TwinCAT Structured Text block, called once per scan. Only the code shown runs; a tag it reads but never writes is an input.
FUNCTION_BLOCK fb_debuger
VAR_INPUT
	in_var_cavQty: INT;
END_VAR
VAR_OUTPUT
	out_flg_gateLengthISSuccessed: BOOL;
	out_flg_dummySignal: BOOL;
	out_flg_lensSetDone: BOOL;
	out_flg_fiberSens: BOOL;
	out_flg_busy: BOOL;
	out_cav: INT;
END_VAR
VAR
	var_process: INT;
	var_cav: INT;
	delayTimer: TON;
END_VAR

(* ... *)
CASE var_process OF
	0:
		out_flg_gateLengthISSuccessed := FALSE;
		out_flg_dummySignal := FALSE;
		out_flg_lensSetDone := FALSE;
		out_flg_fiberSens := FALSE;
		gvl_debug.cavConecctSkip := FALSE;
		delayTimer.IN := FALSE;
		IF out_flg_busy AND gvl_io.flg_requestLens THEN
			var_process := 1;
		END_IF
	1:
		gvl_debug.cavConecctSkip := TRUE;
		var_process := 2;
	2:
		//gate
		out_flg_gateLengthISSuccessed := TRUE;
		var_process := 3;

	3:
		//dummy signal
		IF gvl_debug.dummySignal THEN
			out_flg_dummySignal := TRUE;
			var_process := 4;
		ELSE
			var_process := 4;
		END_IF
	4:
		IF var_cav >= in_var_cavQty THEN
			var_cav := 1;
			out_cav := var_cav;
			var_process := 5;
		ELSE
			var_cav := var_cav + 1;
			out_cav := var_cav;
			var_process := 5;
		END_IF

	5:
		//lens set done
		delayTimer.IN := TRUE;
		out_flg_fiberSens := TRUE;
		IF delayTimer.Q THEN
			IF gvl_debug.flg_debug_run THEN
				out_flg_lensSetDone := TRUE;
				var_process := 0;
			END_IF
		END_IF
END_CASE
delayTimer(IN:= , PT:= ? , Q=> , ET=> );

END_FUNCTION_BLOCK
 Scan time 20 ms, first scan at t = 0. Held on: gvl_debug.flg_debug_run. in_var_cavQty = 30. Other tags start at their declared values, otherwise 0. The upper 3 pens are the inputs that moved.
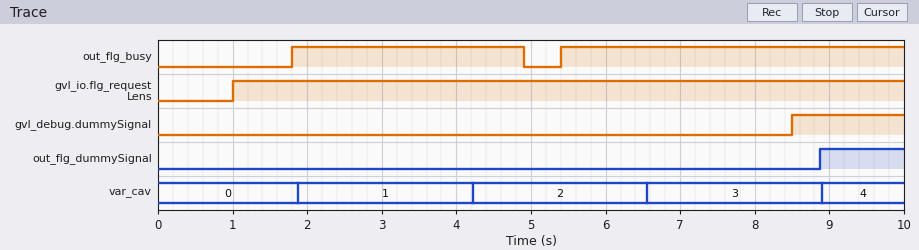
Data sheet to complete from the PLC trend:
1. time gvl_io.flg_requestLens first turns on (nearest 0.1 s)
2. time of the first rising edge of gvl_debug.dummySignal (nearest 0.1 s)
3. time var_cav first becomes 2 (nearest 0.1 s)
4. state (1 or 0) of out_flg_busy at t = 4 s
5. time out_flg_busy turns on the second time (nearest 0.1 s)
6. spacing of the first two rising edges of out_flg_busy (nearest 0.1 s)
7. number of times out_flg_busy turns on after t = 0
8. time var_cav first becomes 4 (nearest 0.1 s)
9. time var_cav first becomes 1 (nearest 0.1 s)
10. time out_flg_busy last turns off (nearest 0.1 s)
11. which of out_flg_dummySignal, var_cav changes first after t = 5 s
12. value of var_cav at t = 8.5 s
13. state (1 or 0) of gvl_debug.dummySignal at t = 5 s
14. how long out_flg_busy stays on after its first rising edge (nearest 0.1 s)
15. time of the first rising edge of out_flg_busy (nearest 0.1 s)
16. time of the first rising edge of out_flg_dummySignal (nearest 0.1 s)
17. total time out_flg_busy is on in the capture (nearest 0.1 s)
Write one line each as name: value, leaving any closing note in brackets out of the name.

time gvl_io.flg_requestLens first turns on: 1.0 s
time of the first rising edge of gvl_debug.dummySignal: 8.5 s
time var_cav first becomes 2: 4.2 s
state (1 or 0) of out_flg_busy at t = 4 s: 1
time out_flg_busy turns on the second time: 5.4 s
spacing of the first two rising edges of out_flg_busy: 3.6 s
number of times out_flg_busy turns on after t = 0: 2
time var_cav first becomes 4: 8.9 s
time var_cav first becomes 1: 1.9 s
time out_flg_busy last turns off: 4.9 s
which of out_flg_dummySignal, var_cav changes first after t = 5 s: var_cav
value of var_cav at t = 8.5 s: 3
state (1 or 0) of gvl_debug.dummySignal at t = 5 s: 0
how long out_flg_busy stays on after its first rising edge: 3.1 s
time of the first rising edge of out_flg_busy: 1.8 s
time of the first rising edge of out_flg_dummySignal: 8.9 s
total time out_flg_busy is on in the capture: 7.7 s
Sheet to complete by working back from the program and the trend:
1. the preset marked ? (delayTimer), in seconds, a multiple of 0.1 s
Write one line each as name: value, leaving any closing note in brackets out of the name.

the preset marked ? (delayTimer), in seconds, a multiple of 0.1 s: 2.2 s
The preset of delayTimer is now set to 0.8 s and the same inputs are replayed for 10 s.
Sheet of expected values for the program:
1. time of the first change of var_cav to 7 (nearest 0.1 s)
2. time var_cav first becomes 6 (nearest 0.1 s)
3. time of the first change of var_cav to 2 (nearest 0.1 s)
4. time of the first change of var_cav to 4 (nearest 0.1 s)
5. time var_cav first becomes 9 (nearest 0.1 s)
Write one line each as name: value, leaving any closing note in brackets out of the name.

time of the first change of var_cav to 7: 7.5 s
time var_cav first becomes 6: 6.6 s
time of the first change of var_cav to 2: 2.8 s
time of the first change of var_cav to 4: 4.7 s
time var_cav first becomes 9: 9.4 s
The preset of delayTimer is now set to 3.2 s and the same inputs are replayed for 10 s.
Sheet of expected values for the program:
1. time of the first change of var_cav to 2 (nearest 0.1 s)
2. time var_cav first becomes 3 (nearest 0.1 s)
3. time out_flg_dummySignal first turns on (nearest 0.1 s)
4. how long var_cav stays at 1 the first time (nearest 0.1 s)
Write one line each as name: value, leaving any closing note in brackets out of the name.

time of the first change of var_cav to 2: 5.5 s
time var_cav first becomes 3: 8.8 s
time out_flg_dummySignal first turns on: 8.8 s
how long var_cav stays at 1 the first time: 3.6 s
